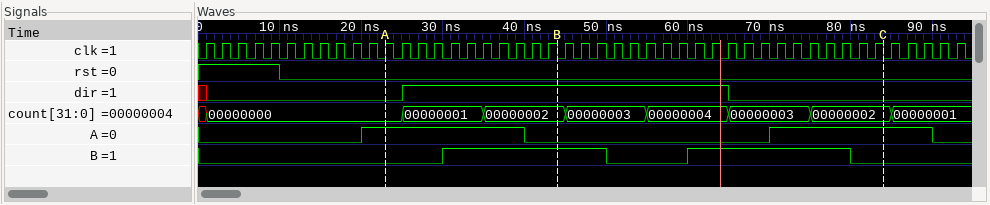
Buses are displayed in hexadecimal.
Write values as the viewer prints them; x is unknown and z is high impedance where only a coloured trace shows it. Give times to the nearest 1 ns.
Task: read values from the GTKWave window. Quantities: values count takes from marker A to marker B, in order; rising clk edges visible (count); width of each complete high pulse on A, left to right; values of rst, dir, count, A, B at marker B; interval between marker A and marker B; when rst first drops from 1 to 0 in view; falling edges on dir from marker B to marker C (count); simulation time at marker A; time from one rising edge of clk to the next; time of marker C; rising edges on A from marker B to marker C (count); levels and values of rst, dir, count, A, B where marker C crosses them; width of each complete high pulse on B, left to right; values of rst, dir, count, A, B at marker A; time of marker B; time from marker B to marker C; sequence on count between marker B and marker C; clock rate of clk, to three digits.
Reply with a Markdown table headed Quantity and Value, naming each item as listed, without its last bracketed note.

| Quantity | Value |
|---|---|
| values count takes from marker A to marker B, in order | 00000000, 00000001, 00000002 |
| rising clk edges visible | 47 |
| width of each complete high pulse on A, left to right | 20 ns, 20 ns |
| values of rst, dir, count, A, B at marker B | rst=0, dir=1, count=00000002, A=0, B=1 |
| interval between marker A and marker B | 21 ns |
| when rst first drops from 1 to 0 in view | 10 ns |
| falling edges on dir from marker B to marker C | 1 |
| simulation time at marker A | 23 ns |
| time from one rising edge of clk to the next | 2 ns |
| time of marker C | 84 ns |
| rising edges on A from marker B to marker C | 1 |
| levels and values of rst, dir, count, A, B where marker C crosses them | rst=0, dir=0, count=00000002, A=1, B=0 |
| width of each complete high pulse on B, left to right | 20 ns, 20 ns |
| values of rst, dir, count, A, B at marker A | rst=0, dir=0, count=00000000, A=1, B=0 |
| time of marker B | 44 ns |
| time from marker B to marker C | 40 ns |
| sequence on count between marker B and marker C | 00000002, 00000003, 00000004, 00000003, 00000002 |
| clock rate of clk, to three digits | 500 MHz |
